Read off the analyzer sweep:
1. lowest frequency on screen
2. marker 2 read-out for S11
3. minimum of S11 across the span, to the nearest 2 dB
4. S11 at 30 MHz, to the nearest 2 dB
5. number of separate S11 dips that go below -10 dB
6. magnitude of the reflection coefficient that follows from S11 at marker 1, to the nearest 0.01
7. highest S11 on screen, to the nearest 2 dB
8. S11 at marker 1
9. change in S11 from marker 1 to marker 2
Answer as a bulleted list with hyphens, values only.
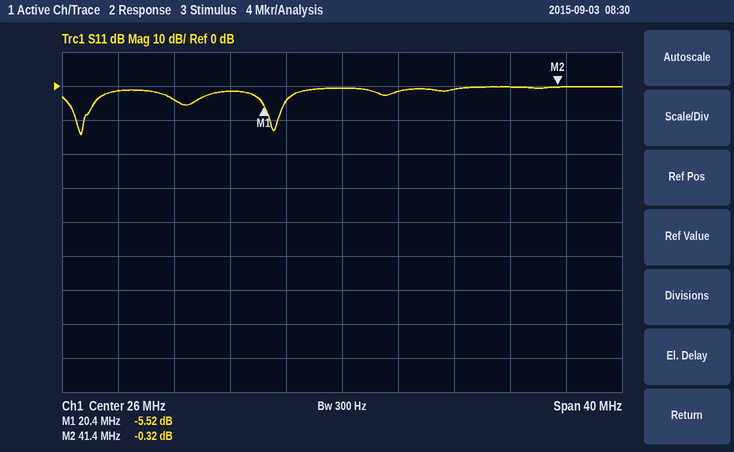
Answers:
- 6 MHz
- -0.32 dB
- -14 dB
- -2 dB
- 2
- 0.53
- 0 dB
- -5.52 dB
- 5.20 dB
